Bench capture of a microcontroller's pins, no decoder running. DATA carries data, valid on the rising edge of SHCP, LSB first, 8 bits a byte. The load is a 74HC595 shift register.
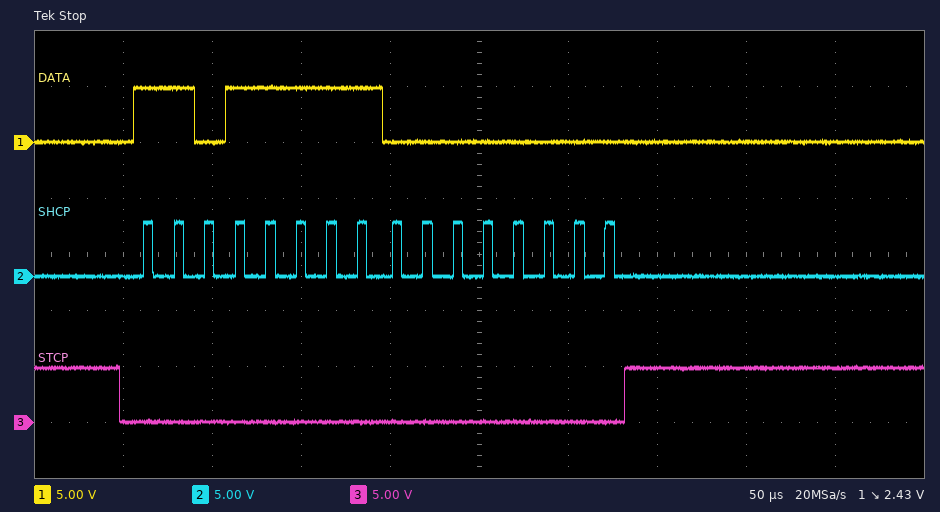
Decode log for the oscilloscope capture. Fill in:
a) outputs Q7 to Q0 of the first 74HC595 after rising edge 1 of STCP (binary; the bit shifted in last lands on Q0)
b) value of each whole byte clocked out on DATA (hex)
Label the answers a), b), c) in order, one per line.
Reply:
a) 00000000
b) FB 00
